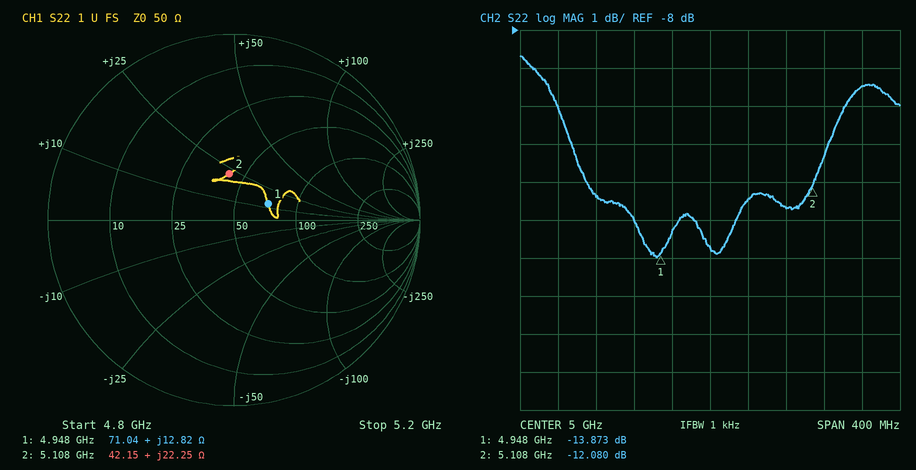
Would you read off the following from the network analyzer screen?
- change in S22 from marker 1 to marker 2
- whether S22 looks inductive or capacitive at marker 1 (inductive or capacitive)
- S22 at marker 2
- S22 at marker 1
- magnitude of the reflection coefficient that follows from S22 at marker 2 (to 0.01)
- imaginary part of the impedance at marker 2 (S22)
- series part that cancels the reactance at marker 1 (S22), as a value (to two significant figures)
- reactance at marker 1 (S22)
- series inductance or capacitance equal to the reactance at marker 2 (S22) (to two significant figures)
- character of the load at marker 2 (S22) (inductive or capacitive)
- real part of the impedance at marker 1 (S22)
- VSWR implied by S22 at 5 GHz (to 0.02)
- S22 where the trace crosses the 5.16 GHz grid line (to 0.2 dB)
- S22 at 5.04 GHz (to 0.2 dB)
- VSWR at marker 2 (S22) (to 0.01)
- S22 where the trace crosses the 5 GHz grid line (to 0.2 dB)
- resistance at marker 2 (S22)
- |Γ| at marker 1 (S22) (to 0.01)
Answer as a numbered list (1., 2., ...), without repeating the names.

1. 1.793 dB
2. inductive
3. -12.080 dB
4. -13.873 dB
5. 0.25
6. +22.25 Ω
7. 2.5 pF
8. +12.82 Ω
9. 690 pH
10. inductive
11. 71.04 Ω
12. 1.52
13. -9.4 dB
14. -12.4 dB
15. 1.66
16. -13.8 dB
17. 42.15 Ω
18. 0.20
